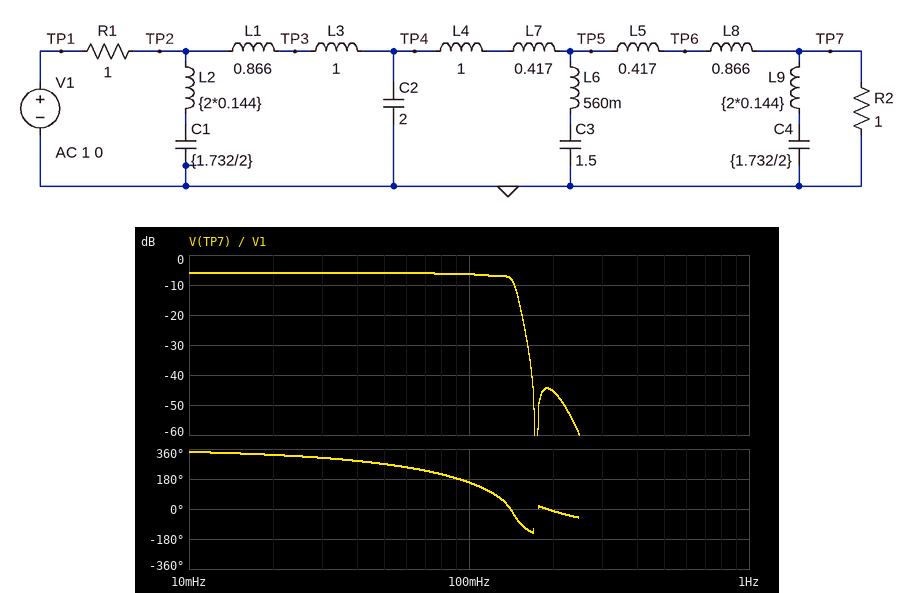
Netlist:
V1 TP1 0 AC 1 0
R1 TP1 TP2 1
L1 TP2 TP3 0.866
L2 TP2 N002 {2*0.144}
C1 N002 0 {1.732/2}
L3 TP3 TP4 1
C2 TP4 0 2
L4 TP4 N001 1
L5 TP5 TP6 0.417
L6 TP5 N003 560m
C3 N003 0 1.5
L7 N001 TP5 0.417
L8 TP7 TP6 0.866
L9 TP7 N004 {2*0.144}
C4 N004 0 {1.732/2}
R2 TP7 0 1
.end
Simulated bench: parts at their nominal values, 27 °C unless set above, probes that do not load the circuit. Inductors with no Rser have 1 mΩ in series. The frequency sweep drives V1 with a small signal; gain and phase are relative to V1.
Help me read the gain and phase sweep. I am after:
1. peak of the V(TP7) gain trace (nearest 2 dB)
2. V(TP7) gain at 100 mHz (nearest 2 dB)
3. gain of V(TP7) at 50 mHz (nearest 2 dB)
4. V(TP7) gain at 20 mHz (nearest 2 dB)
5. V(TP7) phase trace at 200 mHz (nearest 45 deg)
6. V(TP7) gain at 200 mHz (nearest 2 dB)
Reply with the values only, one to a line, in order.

-6 dB
-6 dB
-6 dB
-6 dB
0 deg
-46 dB
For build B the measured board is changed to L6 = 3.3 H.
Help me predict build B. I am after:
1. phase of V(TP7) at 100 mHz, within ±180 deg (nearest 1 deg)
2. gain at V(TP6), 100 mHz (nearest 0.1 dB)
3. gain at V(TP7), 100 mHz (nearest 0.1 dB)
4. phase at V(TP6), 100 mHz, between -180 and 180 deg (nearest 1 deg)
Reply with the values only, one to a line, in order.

-146 deg
-9.4 dB
-8.2 dB
-107 deg
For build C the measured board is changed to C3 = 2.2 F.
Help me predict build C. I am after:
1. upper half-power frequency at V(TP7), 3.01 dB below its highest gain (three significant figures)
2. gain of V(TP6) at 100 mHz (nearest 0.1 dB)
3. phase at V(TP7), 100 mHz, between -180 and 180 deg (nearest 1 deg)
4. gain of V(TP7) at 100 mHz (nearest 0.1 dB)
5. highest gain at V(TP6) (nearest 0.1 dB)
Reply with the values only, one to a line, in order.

104 mHz
-9.8 dB
134 deg
-8.5 dB
-6.0 dB
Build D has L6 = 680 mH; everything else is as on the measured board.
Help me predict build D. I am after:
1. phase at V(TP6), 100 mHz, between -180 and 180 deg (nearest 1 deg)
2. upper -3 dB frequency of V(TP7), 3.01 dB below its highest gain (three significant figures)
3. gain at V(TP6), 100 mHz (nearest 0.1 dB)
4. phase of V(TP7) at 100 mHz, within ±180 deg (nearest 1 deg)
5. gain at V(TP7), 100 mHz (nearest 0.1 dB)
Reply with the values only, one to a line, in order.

-166 deg
133 mHz
-7.9 dB
155 deg
-6.6 dB
